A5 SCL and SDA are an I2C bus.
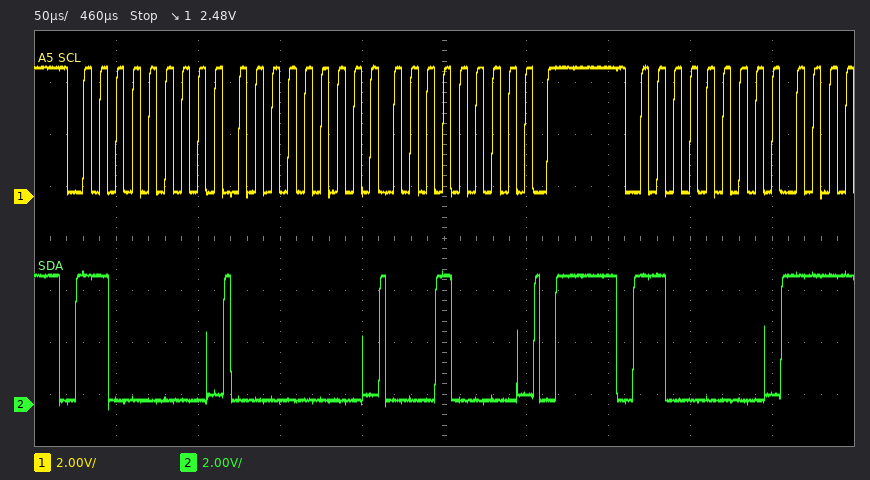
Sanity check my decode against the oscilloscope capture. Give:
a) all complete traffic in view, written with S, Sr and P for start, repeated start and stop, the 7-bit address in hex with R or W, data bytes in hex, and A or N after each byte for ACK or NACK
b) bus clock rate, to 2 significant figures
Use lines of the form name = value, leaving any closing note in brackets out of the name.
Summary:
all complete traffic in view, written with S, Sr and P for start, repeated start and stop, the 7-bit address in hex with R or W, data bytes in hex, and A or N after each byte for ACK or NACK = S 60W A 00 A 10 A P S 60W A
bus clock rate, to 2 significant figures = 100 kHz
